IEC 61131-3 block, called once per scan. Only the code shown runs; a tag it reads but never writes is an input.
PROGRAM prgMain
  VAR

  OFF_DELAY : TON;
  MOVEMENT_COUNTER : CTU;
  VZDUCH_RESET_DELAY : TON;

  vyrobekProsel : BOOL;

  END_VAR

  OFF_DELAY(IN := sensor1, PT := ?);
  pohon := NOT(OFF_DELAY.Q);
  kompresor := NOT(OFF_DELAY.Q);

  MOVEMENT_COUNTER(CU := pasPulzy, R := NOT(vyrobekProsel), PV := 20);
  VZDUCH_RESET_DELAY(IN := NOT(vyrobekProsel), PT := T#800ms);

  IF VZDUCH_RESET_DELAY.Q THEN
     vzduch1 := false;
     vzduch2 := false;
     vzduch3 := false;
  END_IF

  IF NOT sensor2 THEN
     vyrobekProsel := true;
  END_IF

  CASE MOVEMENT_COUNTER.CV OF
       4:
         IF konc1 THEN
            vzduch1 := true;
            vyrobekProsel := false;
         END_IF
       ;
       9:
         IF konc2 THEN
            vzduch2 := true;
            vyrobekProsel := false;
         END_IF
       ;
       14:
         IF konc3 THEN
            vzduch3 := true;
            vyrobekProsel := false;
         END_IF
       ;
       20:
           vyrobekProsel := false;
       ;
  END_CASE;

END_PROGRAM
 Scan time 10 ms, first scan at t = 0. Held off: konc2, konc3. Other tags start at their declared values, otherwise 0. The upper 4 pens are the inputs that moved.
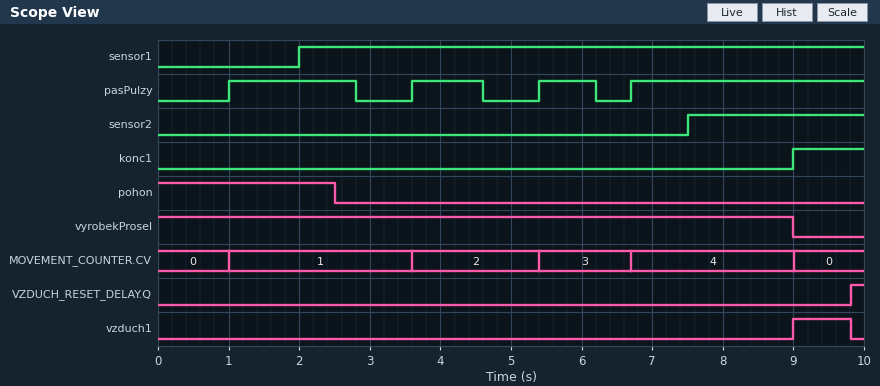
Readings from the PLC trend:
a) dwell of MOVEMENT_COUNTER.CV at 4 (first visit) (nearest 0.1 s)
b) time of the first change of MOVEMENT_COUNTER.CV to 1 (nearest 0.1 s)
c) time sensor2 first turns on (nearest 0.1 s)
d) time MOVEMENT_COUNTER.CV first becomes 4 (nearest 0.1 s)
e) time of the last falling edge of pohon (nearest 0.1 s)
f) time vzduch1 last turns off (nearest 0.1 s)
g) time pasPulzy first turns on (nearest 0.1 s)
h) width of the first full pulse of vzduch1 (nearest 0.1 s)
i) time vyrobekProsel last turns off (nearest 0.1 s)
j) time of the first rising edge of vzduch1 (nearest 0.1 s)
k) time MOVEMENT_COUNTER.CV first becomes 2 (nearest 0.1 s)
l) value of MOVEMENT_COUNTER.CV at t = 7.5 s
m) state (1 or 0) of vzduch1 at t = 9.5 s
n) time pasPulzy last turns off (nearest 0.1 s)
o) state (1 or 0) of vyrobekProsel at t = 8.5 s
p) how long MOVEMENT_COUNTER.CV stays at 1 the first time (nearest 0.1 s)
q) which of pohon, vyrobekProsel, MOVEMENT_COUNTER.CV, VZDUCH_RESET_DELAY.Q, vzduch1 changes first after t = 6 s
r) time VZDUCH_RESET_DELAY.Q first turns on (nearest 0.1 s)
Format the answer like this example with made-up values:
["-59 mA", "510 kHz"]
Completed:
["2.3 s", "1.0 s", "7.5 s", "6.7 s", "2.5 s", "9.8 s", "1.0 s", "0.8 s", "9.0 s", "9.0 s", "3.6 s", "4", "1", "6.2 s", "1", "2.6 s", "MOVEMENT_COUNTER.CV", "9.8 s"]
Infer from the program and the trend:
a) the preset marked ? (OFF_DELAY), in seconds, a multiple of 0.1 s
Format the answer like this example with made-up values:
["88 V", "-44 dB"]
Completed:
["0.5 s"]
